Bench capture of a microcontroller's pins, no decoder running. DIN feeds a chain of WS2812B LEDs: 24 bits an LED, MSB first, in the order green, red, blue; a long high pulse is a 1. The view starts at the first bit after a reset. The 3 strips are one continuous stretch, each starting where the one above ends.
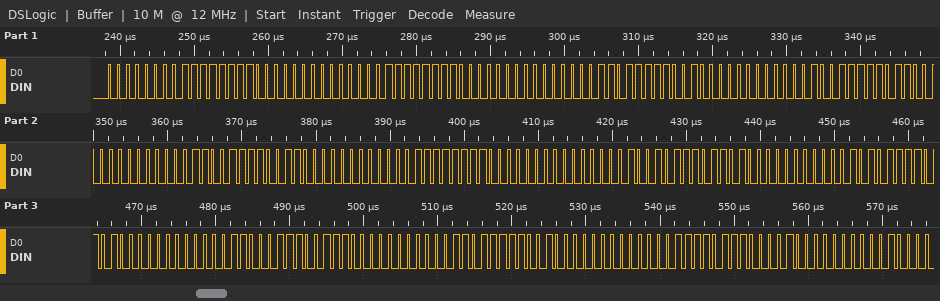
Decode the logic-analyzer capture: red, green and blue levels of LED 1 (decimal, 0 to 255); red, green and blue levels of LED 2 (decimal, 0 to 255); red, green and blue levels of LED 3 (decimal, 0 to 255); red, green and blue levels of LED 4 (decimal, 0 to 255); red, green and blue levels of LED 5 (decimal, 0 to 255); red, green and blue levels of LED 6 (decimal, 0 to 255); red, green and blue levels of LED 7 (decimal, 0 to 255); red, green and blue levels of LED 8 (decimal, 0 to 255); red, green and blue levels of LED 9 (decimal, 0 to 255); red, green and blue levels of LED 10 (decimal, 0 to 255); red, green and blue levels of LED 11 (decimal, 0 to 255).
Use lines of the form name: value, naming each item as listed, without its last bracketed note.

red, green and blue levels of LED 1: 255, 0, 0
red, green and blue levels of LED 2: 252, 3, 0
red, green and blue levels of LED 3: 249, 6, 0
red, green and blue levels of LED 4: 246, 9, 0
red, green and blue levels of LED 5: 243, 12, 0
red, green and blue levels of LED 6: 240, 15, 0
red, green and blue levels of LED 7: 237, 18, 0
red, green and blue levels of LED 8: 234, 21, 0
red, green and blue levels of LED 9: 231, 24, 0
red, green and blue levels of LED 10: 228, 27, 0
red, green and blue levels of LED 11: 225, 30, 0
